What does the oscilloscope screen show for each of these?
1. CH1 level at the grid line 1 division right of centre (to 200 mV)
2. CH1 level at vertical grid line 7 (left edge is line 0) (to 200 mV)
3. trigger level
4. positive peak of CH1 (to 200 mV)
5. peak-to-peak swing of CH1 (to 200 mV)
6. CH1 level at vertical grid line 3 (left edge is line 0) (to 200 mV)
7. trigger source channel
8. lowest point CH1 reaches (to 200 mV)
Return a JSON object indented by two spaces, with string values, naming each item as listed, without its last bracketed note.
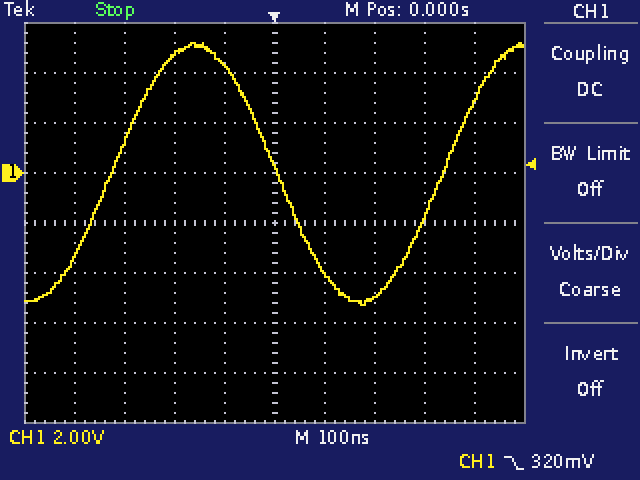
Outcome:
{
  "CH1 level at the grid line 1 division right of centre": "-4.0 V",
  "CH1 level at vertical grid line 7 (left edge is line 0)": "-5.0 V",
  "trigger level": "320 mV",
  "positive peak of CH1": "5.2 V",
  "peak-to-peak swing of CH1": "10.4 V",
  "CH1 level at vertical grid line 3 (left edge is line 0)": "4.8 V",
  "trigger source channel": "CH1",
  "lowest point CH1 reaches": "-5.2 V"
}
